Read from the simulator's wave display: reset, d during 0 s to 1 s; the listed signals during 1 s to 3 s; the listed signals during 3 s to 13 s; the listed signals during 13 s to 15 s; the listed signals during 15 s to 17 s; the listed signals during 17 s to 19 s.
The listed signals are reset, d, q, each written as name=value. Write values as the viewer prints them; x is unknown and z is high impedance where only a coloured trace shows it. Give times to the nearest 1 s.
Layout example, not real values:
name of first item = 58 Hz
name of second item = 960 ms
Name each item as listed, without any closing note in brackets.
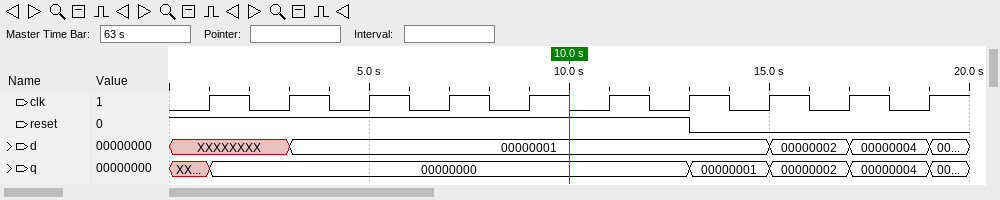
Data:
reset, d during 0 s to 1 s = reset=1, d=XXXXXXXX
the listed signals during 1 s to 3 s = reset=1, d=XXXXXXXX, q=00000000
the listed signals during 3 s to 13 s = reset=1, d=00000001, q=00000000
the listed signals during 13 s to 15 s = reset=0, d=00000001, q=00000001
the listed signals during 15 s to 17 s = reset=0, d=00000002, q=00000002
the listed signals during 17 s to 19 s = reset=0, d=00000004, q=00000004
